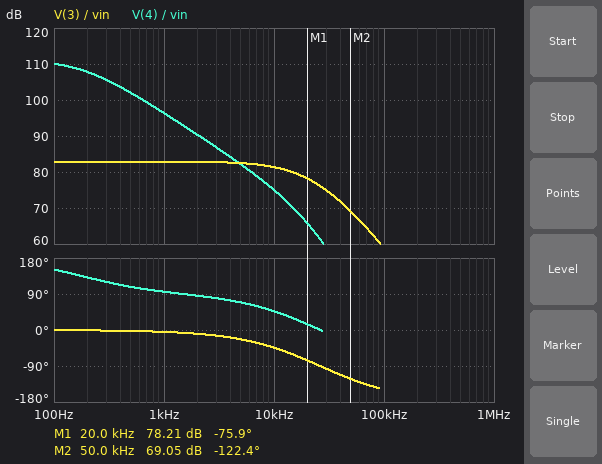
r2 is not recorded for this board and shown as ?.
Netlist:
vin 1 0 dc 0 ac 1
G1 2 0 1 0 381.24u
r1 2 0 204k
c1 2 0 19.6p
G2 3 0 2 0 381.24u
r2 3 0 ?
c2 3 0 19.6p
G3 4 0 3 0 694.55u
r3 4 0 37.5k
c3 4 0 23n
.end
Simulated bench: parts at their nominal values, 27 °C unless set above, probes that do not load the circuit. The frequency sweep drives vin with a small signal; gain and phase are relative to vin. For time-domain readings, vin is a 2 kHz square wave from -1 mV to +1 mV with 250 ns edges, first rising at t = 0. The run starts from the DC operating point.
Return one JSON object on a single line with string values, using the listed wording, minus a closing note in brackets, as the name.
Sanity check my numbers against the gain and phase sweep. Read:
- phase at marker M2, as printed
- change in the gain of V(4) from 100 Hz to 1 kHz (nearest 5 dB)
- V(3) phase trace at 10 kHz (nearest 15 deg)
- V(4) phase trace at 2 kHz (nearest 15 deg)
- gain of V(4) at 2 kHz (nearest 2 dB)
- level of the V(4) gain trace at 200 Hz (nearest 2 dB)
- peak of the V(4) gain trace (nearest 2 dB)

{"phase at marker M2, as printed": "-122.4 deg", "change in the gain of V(4) from 100 Hz to 1 kHz": "-15 dB", "V(3) phase trace at 10 kHz": "-45 deg", "V(4) phase trace at 2 kHz": "90 deg", "gain of V(4) at 2 kHz": "90 dB", "level of the V(4) gain trace at 200 Hz": "108 dB", "peak of the V(4) gain trace": "110 dB"}
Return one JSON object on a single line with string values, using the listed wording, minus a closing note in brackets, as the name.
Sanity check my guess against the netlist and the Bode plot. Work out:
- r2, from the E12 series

{"r2, from the E12 series": "470 kΩ"}
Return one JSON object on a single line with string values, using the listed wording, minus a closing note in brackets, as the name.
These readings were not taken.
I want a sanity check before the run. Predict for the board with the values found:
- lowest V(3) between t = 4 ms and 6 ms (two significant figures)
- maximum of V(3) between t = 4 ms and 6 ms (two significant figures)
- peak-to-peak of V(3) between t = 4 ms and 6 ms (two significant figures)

{"lowest V(3) between t = 4 ms and 6 ms": "-14 V", "maximum of V(3) between t = 4 ms and 6 ms": "14 V", "peak-to-peak of V(3) between t = 4 ms and 6 ms": "28 V"}
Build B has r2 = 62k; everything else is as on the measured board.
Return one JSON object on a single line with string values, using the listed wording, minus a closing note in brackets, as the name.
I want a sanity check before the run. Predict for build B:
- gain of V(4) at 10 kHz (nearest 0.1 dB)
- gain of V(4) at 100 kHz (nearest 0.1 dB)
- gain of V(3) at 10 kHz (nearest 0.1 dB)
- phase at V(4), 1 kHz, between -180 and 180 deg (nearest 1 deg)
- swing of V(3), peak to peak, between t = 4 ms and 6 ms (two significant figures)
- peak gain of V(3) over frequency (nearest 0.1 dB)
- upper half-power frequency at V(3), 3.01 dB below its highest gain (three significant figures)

{"gain of V(4) at 10 kHz": "58.6 dB", "gain of V(4) at 100 kHz": "28.3 dB", "gain of V(3) at 10 kHz": "65.0 dB", "phase at V(4), 1 kHz, between -180 and 180 deg": "99 deg", "swing of V(3), peak to peak, between t = 4 ms and 6 ms": "3.7 V", "peak gain of V(3) over frequency": "65.3 dB", "upper half-power frequency at V(3), 3.01 dB below its highest gain": "36.8 kHz"}
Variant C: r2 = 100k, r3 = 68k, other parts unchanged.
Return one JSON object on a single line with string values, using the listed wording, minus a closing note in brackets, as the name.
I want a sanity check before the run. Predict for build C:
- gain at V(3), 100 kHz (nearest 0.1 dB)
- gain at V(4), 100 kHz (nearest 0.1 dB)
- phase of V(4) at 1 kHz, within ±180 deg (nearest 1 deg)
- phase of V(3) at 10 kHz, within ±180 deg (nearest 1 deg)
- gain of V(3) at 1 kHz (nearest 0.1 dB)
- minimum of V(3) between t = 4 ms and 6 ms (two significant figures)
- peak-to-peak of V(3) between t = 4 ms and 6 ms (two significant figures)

{"gain at V(3), 100 kHz": "56.8 dB", "gain at V(4), 100 kHz": "30.4 dB", "phase of V(4) at 1 kHz, within ±180 deg": "94 deg", "phase of V(3) at 10 kHz, within ±180 deg": "-21 deg", "gain of V(3) at 1 kHz": "69.4 dB", "minimum of V(3) between t = 4 ms and 6 ms": "-3.0 V", "peak-to-peak of V(3) between t = 4 ms and 6 ms": "5.9 V"}
